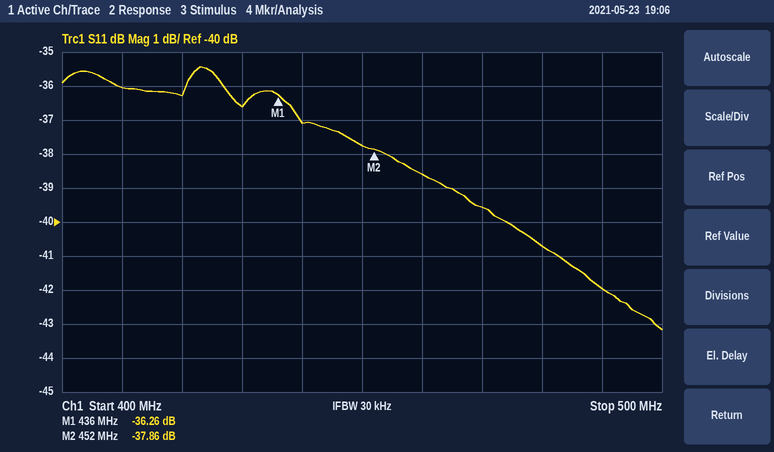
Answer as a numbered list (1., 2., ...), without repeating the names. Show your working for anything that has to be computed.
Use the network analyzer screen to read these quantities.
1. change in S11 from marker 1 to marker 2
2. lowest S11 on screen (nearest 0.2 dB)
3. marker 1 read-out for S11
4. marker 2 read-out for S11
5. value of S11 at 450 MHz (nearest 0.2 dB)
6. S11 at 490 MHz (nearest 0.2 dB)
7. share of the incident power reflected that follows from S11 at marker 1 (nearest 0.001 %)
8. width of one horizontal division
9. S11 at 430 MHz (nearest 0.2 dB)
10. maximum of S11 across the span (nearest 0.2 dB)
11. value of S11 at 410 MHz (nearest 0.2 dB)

1. -37.86 − (-36.26) = -1.60 dB
2. -43.2 dB
3. -36.26 dB
4. -37.86 dB
5. -37.8 dB
6. -42.0 dB
7. 10^(-36.26/10) ≈ 0.024 %
8. 10 MHz
9. -36.6 dB
10. -35.4 dB
11. -36.0 dB
